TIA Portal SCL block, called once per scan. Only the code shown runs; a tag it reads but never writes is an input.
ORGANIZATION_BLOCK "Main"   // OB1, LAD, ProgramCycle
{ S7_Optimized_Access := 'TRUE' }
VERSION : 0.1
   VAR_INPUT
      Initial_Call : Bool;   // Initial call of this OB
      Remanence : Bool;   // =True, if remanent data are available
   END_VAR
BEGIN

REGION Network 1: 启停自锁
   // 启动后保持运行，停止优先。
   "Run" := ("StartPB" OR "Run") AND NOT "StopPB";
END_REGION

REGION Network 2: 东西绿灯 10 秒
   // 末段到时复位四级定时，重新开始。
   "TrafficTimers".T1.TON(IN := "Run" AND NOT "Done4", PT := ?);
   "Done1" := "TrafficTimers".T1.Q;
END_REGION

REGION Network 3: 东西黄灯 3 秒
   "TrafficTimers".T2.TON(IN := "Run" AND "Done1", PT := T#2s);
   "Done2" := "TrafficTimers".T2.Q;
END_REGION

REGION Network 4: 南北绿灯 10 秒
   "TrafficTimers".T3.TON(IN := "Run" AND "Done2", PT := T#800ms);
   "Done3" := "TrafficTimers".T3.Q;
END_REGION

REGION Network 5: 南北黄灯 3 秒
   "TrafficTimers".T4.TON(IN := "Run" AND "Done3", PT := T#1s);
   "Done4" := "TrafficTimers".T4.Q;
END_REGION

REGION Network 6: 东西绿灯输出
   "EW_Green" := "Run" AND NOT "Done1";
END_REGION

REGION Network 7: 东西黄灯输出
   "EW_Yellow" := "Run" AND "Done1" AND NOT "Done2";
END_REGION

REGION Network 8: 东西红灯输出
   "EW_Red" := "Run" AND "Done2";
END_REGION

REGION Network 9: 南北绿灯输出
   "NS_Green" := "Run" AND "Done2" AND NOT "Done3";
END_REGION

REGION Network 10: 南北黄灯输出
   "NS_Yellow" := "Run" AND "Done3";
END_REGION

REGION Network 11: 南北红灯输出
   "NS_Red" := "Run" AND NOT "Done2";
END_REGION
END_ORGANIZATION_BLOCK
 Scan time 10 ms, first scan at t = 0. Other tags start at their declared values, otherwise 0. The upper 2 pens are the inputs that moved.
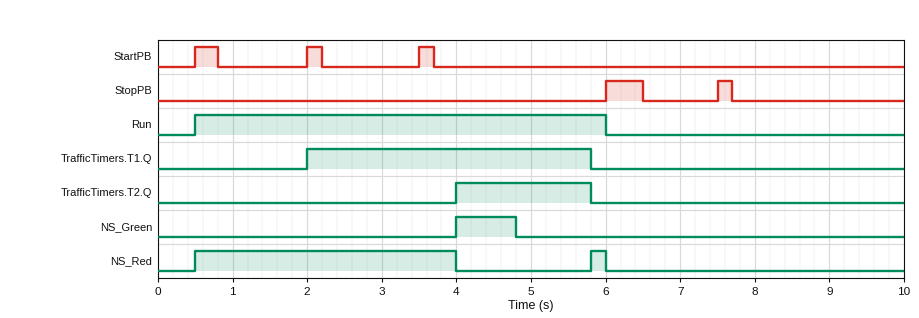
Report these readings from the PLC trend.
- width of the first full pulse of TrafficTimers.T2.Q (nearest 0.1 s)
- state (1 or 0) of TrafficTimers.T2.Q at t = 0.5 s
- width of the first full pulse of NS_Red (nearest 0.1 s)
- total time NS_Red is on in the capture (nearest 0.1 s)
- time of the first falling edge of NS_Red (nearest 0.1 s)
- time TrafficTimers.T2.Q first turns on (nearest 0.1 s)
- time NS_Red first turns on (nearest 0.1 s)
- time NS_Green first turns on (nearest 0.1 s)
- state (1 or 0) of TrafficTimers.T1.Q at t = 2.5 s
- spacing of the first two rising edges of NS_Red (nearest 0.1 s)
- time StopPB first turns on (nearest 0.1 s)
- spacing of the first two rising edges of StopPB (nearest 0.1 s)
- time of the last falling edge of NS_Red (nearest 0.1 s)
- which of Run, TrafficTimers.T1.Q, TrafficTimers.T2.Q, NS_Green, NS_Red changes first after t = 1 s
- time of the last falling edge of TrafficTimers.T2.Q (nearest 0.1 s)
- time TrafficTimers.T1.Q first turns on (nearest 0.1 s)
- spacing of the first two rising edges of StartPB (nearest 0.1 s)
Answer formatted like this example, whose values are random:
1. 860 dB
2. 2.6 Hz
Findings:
1. 1.8 s
2. 0
3. 3.5 s
4. 3.7 s
5. 4.0 s
6. 4.0 s
7. 0.5 s
8. 4.0 s
9. 1
10. 5.3 s
11. 6.0 s
12. 1.5 s
13. 6.0 s
14. TrafficTimers.T1.Q
15. 5.8 s
16. 2.0 s
17. 1.5 s
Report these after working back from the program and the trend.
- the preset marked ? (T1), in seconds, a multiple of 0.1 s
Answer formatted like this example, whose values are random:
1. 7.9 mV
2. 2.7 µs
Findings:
1. 1.5 s
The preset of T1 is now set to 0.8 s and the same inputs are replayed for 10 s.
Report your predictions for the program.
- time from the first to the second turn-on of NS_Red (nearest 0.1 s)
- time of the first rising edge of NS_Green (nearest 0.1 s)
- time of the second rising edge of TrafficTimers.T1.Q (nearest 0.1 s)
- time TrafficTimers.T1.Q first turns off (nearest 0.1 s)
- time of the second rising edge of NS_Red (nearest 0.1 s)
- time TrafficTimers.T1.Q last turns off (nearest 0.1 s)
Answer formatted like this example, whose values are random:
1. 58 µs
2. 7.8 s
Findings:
1. 4.6 s
2. 3.3 s
3. 5.9 s
4. 5.1 s
5. 5.1 s
6. 6.0 s
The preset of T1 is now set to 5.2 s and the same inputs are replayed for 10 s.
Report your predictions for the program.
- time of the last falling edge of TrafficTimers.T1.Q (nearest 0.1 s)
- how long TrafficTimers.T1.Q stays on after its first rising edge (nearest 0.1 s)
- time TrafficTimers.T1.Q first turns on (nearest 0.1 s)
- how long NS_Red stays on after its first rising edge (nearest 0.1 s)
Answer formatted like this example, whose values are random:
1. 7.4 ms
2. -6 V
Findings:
1. 6.0 s
2. 0.3 s
3. 5.7 s
4. 5.5 s
